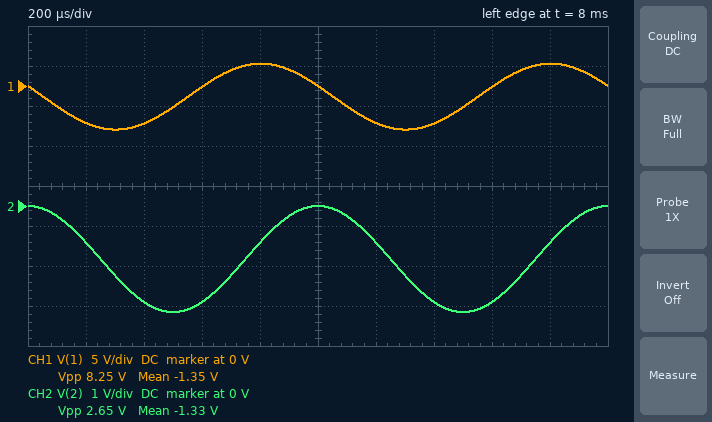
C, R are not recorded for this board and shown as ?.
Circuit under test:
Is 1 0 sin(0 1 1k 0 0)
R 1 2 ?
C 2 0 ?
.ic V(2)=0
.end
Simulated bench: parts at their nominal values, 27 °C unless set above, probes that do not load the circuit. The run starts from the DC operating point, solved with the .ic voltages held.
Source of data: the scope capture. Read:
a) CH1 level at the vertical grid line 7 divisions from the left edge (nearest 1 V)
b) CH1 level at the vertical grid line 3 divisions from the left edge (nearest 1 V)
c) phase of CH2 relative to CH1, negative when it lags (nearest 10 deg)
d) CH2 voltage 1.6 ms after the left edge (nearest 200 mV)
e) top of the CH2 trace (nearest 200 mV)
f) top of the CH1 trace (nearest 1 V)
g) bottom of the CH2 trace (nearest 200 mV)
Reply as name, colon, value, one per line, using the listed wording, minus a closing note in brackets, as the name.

CH1 level at the vertical grid line 7 divisions from the left edge: -5 V
CH1 level at the vertical grid line 3 divisions from the left edge: 0 V
phase of CH2 relative to CH1, negative when it lags: -70 deg
CH2 voltage 1.6 ms after the left edge: -2.4 V
top of the CH2 trace: 0 V
top of the CH1 trace: 3 V
bottom of the CH2 trace: -2.6 V
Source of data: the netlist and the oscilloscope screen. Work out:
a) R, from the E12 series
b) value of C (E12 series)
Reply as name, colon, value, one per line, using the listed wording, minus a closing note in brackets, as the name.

R, from the E12 series: 3.9 Ω
value of C: 120 µF
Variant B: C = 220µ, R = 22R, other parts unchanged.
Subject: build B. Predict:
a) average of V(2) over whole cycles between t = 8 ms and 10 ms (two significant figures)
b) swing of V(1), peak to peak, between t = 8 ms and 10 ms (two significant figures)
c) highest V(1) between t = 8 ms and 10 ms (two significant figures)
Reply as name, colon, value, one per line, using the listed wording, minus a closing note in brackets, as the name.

average of V(2) over whole cycles between t = 8 ms and 10 ms: -720 mV
swing of V(1), peak to peak, between t = 8 ms and 10 ms: 44 V
highest V(1) between t = 8 ms and 10 ms: 21 V
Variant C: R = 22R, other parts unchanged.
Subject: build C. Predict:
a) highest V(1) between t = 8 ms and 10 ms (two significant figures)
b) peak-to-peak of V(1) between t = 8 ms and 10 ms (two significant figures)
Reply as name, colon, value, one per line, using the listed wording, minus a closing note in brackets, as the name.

highest V(1) between t = 8 ms and 10 ms: 21 V
peak-to-peak of V(1) between t = 8 ms and 10 ms: 44 V
